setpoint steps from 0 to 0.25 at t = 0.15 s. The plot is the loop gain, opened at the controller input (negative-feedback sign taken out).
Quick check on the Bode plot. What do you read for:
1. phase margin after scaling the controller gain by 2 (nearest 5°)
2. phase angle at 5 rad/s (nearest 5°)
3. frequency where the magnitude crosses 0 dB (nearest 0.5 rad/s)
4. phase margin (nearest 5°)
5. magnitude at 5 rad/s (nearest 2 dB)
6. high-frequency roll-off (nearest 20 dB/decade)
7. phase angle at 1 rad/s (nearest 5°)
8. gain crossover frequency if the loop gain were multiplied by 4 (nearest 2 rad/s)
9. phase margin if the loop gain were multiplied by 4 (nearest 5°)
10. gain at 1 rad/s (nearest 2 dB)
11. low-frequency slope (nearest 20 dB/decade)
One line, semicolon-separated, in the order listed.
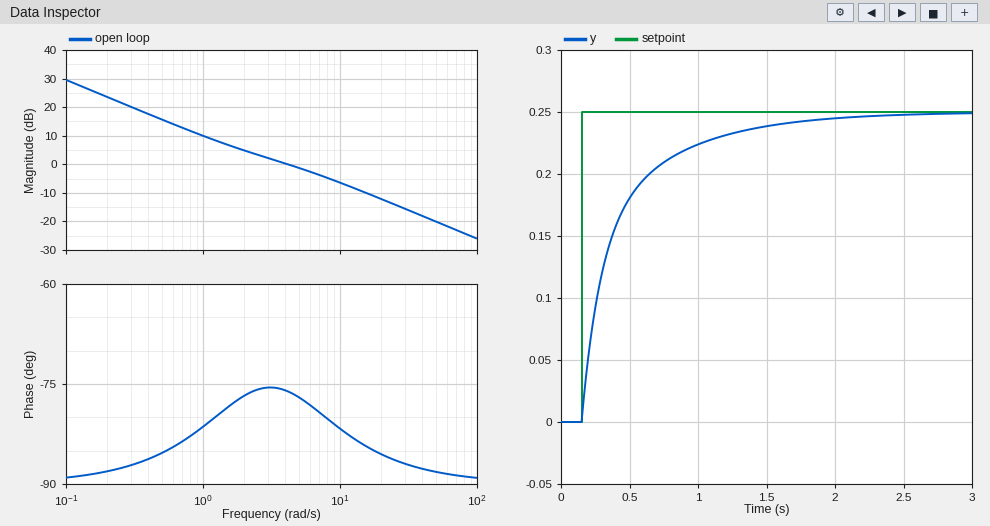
100°; -75°; 4.0 rad/s; 105°; -2 dB; -20 dB/decade; -80°; 20 rad/s; 95°; 10 dB; -20 dB/decade
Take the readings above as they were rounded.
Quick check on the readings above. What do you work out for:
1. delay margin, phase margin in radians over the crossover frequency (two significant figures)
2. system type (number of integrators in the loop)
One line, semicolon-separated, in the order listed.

0.46 s; 1
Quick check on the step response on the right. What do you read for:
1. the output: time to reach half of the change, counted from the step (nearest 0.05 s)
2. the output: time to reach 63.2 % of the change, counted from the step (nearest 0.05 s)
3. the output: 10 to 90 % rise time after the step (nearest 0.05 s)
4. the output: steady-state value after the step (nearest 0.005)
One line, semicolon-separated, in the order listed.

0.15 s; 0.25 s; 0.85 s; 0.250
